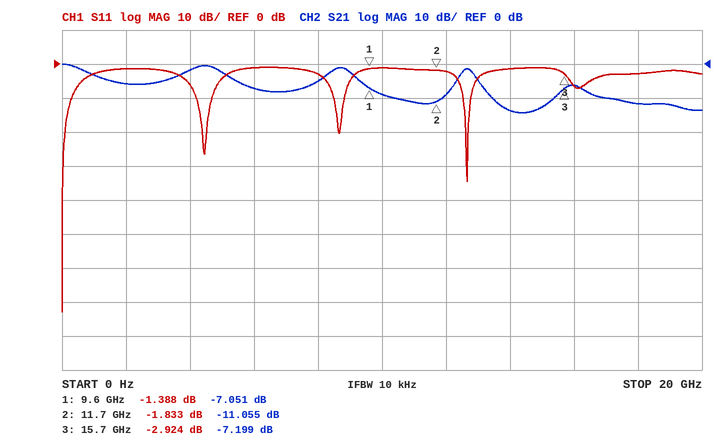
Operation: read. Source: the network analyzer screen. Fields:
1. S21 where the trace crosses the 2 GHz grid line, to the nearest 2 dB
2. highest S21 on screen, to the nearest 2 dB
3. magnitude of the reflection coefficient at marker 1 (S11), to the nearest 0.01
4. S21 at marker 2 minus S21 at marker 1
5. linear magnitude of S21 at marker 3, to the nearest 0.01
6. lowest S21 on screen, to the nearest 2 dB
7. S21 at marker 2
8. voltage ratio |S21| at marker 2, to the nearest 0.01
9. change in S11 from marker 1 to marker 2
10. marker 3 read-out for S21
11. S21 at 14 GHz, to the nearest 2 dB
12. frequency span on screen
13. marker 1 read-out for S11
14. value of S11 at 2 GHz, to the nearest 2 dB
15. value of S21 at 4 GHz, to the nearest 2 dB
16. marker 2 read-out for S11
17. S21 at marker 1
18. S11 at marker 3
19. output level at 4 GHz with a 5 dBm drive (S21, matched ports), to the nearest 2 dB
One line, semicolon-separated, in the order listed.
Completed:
-6 dB; 0 dB; 0.85; -4.004 dB; 0.44; -14 dB; -11.055 dB; 0.28; -0.445 dB; -7.199 dB; -14 dB; 20 GHz; -1.388 dB; -2 dB; -2 dB; -1.833 dB; -7.051 dB; -2.924 dB; 4 dBm
